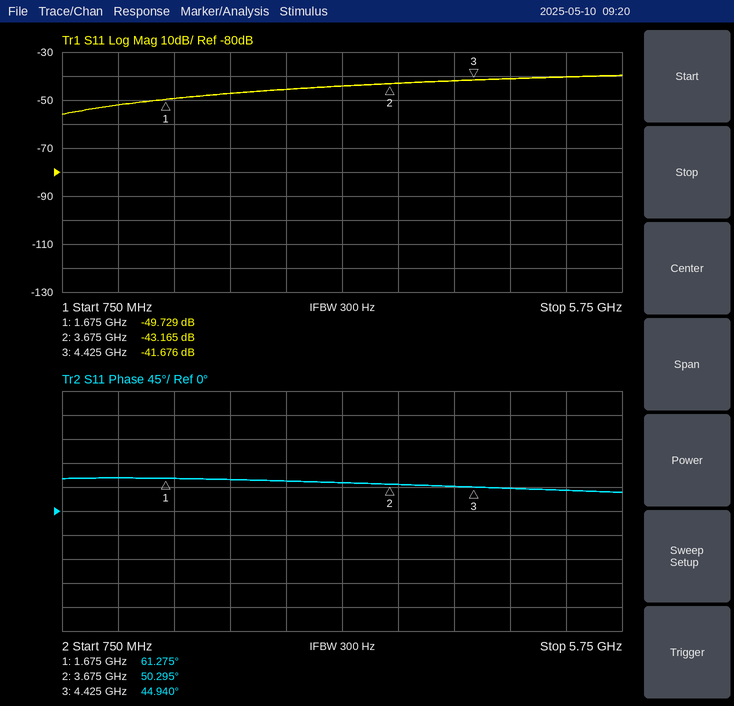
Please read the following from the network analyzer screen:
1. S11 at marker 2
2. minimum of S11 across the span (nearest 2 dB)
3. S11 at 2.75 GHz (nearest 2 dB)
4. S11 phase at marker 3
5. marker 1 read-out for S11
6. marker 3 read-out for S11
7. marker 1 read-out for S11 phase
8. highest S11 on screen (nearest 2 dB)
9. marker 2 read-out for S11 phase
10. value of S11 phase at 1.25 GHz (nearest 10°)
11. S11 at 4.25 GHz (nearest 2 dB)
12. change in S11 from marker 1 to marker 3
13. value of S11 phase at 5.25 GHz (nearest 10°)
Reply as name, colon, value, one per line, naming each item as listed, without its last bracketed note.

S11 at marker 2: -43.165 dB
minimum of S11 across the span: -56 dB
S11 at 2.75 GHz: -46 dB
S11 phase at marker 3: 44.940°
marker 1 read-out for S11: -49.729 dB
marker 3 read-out for S11: -41.676 dB
marker 1 read-out for S11 phase: 61.275°
highest S11 on screen: -40 dB
marker 2 read-out for S11 phase: 50.295°
value of S11 phase at 1.25 GHz: 60°
S11 at 4.25 GHz: -42 dB
change in S11 from marker 1 to marker 3: 8.053 dB
value of S11 phase at 5.25 GHz: 40°
